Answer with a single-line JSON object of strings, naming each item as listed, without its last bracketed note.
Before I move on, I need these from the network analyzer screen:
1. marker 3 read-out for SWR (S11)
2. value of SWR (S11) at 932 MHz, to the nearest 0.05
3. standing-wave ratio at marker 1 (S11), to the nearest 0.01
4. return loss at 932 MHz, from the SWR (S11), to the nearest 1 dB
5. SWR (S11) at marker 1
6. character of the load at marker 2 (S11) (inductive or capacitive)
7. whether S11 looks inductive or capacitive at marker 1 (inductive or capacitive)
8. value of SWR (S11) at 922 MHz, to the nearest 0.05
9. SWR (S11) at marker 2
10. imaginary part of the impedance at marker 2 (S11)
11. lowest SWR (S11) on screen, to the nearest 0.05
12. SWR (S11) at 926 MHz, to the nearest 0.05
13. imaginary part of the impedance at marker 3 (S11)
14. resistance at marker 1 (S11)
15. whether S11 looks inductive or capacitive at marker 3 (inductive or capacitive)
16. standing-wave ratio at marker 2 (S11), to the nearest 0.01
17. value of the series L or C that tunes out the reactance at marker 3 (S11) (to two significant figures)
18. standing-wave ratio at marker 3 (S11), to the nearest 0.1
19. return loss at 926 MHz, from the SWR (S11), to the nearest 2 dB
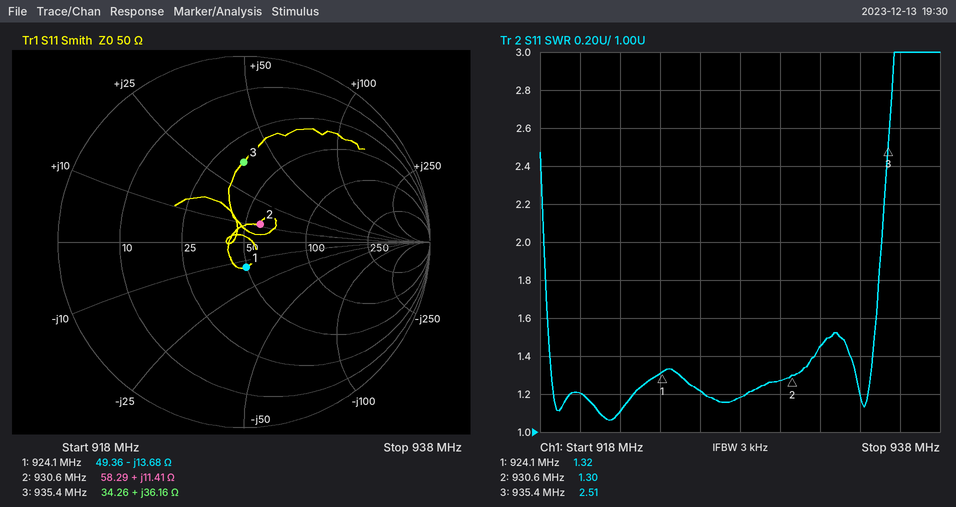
{"marker 3 read-out for SWR": "2.51", "value of SWR (S11) at 932 MHz, to the nearest 0.05": "1.45", "standing-wave ratio at marker 1 (S11), to the nearest 0.01": "1.32", "return loss at 932 MHz, from the SWR (S11), to the nearest 1 dB": "15 dB", "SWR (S11) at marker 1": "1.32", "character of the load at marker 2 (S11)": "inductive", "whether S11 looks inductive or capacitive at marker 1": "capacitive", "value of SWR (S11) at 922 MHz, to the nearest 0.05": "1.10", "SWR (S11) at marker 2": "1.30", "imaginary part of the impedance at marker 2": "+11.41 Ω", "lowest SWR (S11) on screen, to the nearest 0.05": "1.05", "SWR (S11) at 926 MHz, to the nearest 0.05": "1.20", "imaginary part of the impedance at marker 3": "+36.16 Ω", "resistance at marker 1": "49.36 Ω", "whether S11 looks inductive or capacitive at marker 3": "inductive", "standing-wave ratio at marker 2 (S11), to the nearest 0.01": "1.30", "value of the series L or C that tunes out the reactance at marker 3 (S11)": "4.7 pF", "standing-wave ratio at marker 3 (S11), to the nearest 0.1": "2.5", "return loss at 926 MHz, from the SWR (S11), to the nearest 2 dB": "20 dB"}
